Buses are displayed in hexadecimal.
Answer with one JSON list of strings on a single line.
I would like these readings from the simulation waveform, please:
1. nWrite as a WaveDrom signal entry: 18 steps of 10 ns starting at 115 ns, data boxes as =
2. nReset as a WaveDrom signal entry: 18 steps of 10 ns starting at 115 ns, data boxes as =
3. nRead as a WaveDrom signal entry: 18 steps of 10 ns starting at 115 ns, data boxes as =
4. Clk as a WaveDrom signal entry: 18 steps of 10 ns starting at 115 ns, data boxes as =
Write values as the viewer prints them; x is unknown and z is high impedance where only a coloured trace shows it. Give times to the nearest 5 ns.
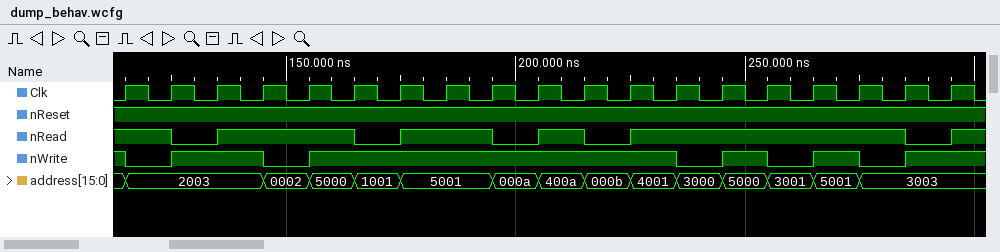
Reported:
["{name: 'nWrite', wave: '01.01.......010101'}", "{name: 'nReset', wave: '1.................'}", "{name: 'nRead', wave: '101..01.0101.....0'}", "{name: 'Clk', wave: 'p.................'}"]
